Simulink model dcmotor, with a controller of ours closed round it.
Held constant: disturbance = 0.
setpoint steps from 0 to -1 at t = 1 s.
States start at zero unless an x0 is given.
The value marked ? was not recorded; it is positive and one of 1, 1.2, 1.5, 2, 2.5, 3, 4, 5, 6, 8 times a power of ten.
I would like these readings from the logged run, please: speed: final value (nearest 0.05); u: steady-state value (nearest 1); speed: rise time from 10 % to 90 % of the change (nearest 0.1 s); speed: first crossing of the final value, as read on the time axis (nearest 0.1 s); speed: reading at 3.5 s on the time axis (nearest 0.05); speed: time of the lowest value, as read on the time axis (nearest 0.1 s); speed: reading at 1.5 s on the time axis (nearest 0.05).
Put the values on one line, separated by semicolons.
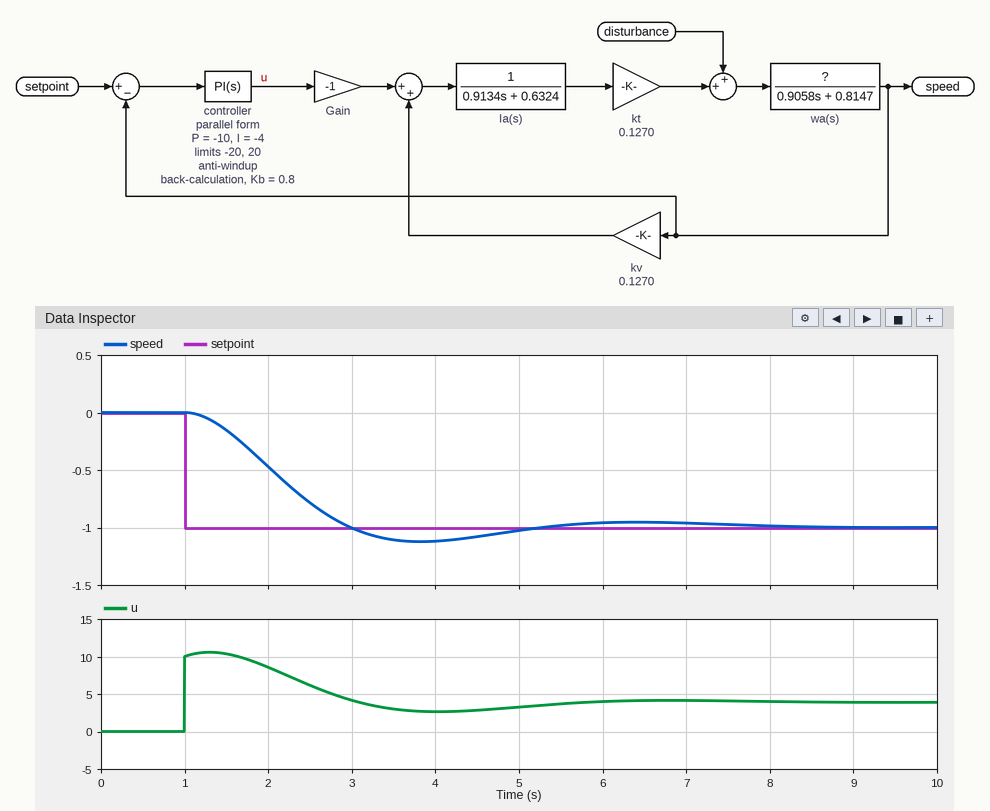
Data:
-1.00; 4; 1.3 s; 3.0 s; -1.10; 3.8 s; -0.15
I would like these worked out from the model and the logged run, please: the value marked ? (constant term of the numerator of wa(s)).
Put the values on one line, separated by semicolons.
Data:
1
